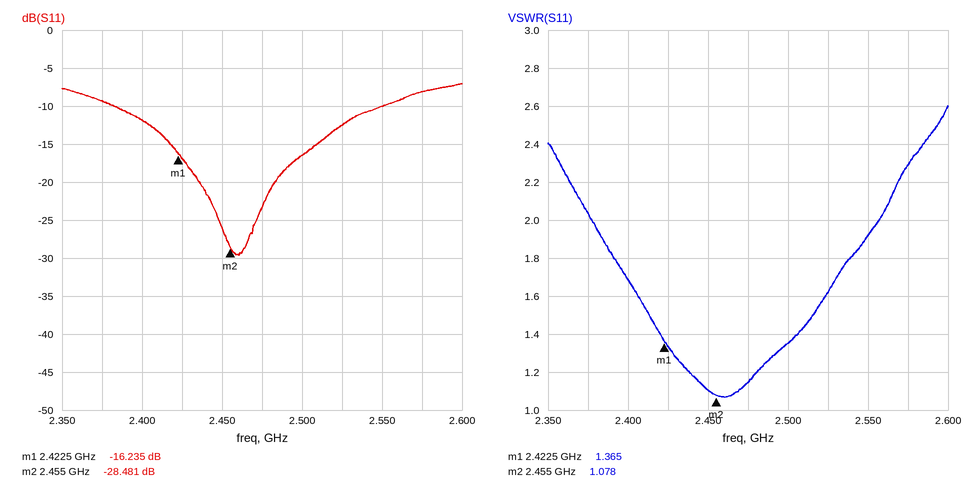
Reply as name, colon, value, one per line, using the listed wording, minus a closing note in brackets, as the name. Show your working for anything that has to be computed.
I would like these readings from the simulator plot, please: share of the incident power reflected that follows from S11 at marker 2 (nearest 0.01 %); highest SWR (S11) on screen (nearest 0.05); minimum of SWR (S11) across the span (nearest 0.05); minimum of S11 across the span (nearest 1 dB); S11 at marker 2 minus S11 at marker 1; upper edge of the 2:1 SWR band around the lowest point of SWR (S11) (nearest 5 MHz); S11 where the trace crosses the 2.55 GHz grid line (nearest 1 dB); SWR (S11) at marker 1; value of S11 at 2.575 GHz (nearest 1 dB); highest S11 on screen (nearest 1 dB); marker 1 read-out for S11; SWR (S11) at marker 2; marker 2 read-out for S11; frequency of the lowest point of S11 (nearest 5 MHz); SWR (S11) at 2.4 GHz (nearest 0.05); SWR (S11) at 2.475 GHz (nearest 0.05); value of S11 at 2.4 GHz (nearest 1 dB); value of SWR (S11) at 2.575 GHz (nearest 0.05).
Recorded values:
share of the incident power reflected that follows from S11 at marker 2: 10^(-28.481/10) ≈ 0.14 %
highest SWR (S11) on screen: 2.60
minimum of SWR (S11) across the span: 1.05
minimum of S11 across the span: -30 dB
S11 at marker 2 minus S11 at marker 1: -28.481 − (-16.235) = -12.246 dB
upper edge of the 2:1 SWR band around the lowest point of SWR (S11): 2.555 GHz
S11 where the trace crosses the 2.55 GHz grid line: -10 dB
SWR (S11) at marker 1: 1.365
value of S11 at 2.575 GHz: -8 dB
highest S11 on screen: -7 dB
marker 1 read-out for S11: -16.235 dB
SWR (S11) at marker 2: 1.078
marker 2 read-out for S11: -28.481 dB
frequency of the lowest point of S11: 2.460 GHz
SWR (S11) at 2.4 GHz: 1.70
SWR (S11) at 2.475 GHz: 1.15
value of S11 at 2.4 GHz: -12 dB
value of SWR (S11) at 2.575 GHz: 2.30
